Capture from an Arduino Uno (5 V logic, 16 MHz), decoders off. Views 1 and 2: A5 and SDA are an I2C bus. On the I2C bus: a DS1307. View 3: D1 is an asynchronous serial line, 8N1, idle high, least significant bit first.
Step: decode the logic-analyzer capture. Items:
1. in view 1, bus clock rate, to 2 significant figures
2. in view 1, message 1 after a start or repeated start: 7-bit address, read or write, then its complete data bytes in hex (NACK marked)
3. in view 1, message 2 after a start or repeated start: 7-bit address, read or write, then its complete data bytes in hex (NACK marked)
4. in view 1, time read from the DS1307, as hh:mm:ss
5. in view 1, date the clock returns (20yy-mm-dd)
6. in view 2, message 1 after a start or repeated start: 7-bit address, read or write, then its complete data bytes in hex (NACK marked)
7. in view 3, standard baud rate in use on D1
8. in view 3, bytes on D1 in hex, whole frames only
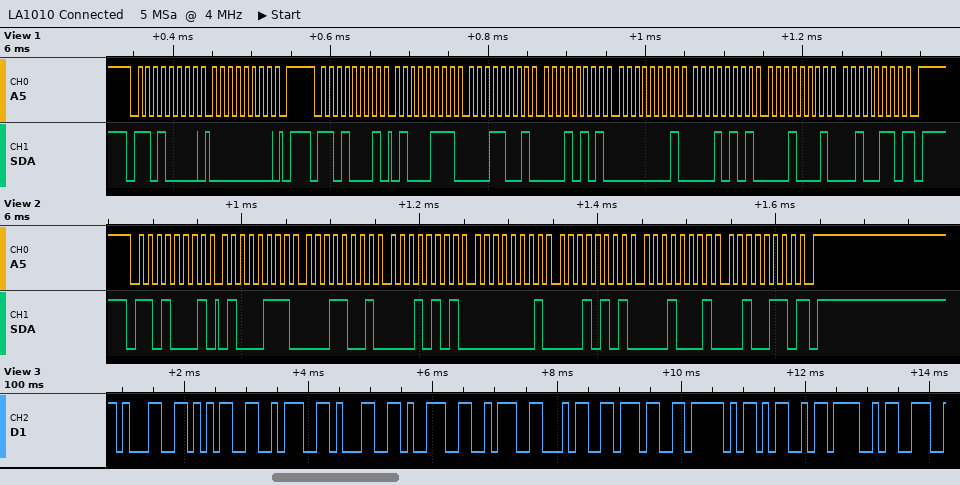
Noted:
100 kHz
0x68 write: 00
0x68 read: 47 19 15 01 15 11 26 NACK
15:19:47
2026-11-15
0x68 read: 47 19 15 01 15 11 26 NACK
9600 baud
31 35 3A 31 39 3A 34 37 5F 4D 4F
